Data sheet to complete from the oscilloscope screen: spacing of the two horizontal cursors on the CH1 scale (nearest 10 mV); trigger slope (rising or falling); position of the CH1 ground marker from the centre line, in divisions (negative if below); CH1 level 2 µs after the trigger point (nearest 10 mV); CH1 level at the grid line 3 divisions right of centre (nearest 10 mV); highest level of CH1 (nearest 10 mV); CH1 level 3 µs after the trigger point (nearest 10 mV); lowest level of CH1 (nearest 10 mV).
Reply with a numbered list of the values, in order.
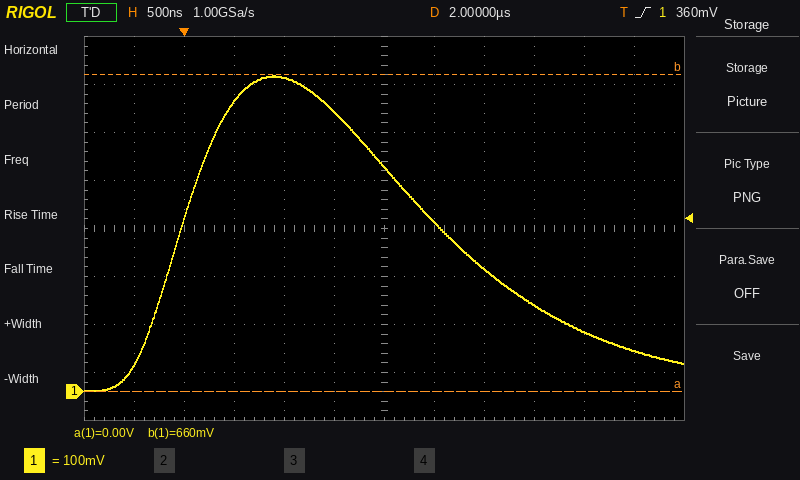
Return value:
1. 660 mV
2. rising
3. -3.4 div
4. 470 mV
5. 180 mV
6. 660 mV
7. 260 mV
8. 0 mV
